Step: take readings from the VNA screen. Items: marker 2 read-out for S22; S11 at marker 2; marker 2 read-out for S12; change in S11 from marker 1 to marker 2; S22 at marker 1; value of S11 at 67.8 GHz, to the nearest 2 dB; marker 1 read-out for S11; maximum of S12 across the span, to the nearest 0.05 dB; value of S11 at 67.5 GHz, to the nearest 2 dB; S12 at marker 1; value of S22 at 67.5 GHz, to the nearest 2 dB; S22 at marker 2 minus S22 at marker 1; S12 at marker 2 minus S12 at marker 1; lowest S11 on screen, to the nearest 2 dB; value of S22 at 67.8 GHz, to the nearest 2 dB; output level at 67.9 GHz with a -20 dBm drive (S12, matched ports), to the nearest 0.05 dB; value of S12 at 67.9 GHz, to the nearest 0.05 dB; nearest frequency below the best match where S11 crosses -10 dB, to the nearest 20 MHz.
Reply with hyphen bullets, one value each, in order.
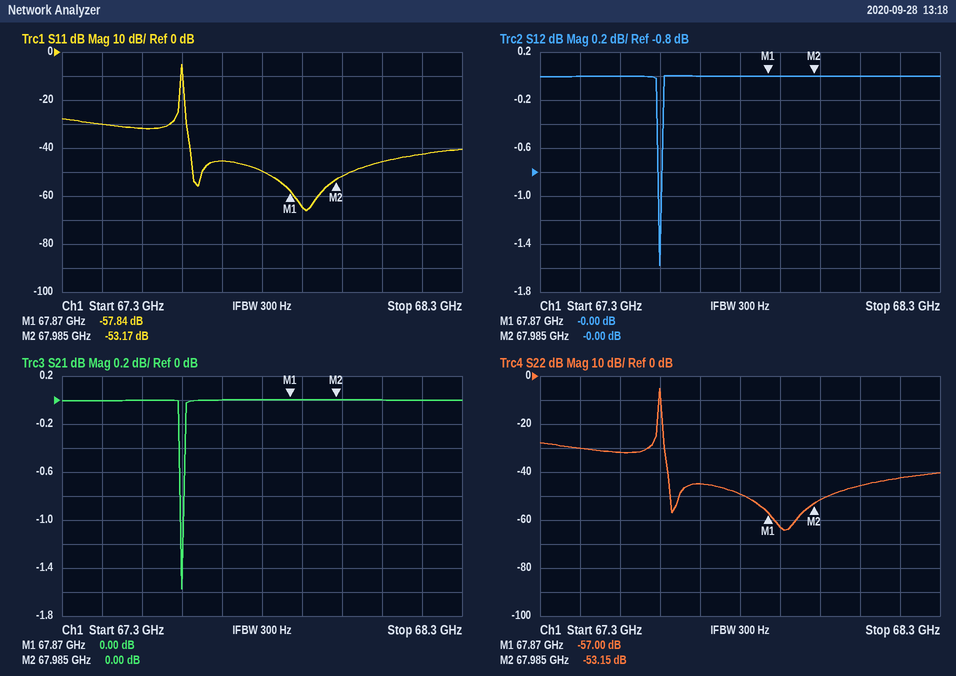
- -53.15 dB
- -53.17 dB
- -0.00 dB
- 4.67 dB
- -57.00 dB
- -50 dB
- -57.84 dB
- 0.00 dB
- -32 dB
- -0.00 dB
- -32 dB
- 3.85 dB
- 0.00 dB
- -66 dB
- -50 dB
- -20.00 dBm
- 0.00 dB
- 67.60 GHz
